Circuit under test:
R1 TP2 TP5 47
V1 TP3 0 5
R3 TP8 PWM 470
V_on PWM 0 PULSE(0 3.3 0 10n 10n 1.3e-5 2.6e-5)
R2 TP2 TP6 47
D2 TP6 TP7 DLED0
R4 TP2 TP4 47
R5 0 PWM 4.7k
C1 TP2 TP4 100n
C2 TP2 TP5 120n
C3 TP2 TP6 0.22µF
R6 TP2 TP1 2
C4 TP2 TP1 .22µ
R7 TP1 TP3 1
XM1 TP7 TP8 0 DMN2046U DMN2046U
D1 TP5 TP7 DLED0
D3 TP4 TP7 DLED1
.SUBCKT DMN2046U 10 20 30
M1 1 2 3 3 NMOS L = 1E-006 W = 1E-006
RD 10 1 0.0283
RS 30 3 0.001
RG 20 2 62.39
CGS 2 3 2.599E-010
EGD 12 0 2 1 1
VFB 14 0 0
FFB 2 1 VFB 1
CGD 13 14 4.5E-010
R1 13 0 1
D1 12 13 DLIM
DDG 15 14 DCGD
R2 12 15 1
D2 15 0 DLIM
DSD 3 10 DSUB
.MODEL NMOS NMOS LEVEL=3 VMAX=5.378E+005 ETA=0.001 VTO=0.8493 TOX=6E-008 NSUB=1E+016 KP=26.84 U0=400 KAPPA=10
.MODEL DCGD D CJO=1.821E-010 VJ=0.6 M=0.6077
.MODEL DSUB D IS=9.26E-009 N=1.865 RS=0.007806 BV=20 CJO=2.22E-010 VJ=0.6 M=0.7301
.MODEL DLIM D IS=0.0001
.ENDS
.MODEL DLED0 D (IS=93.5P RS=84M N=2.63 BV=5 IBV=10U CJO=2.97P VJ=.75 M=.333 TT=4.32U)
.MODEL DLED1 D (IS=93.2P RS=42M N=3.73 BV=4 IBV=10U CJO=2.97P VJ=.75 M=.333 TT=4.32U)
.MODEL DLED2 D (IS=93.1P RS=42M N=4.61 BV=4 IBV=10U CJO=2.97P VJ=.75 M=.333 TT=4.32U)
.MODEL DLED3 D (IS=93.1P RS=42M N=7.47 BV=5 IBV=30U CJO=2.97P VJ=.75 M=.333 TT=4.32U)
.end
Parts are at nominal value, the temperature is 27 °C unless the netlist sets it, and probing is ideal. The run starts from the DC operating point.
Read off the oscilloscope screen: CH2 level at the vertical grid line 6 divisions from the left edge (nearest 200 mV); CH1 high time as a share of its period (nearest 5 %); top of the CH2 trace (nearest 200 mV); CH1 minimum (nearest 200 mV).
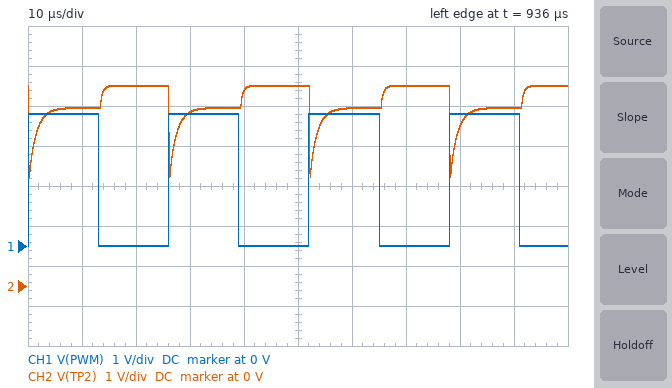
4.4 V
50 %
5.0 V
0 V
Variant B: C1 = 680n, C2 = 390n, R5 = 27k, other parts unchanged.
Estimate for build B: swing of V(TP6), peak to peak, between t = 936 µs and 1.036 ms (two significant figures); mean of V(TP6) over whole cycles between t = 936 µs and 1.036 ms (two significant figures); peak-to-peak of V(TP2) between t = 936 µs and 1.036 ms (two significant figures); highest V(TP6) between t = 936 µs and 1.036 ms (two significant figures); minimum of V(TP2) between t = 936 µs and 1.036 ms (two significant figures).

2.3 V
2.1 V
1.8 V
3.7 V
3.2 V
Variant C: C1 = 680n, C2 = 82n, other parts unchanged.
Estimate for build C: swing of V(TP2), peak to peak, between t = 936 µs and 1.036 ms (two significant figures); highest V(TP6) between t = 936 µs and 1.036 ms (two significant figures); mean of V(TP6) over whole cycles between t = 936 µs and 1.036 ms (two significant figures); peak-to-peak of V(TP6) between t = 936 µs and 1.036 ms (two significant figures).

2.1 V
4.2 V
2.3 V
2.8 V
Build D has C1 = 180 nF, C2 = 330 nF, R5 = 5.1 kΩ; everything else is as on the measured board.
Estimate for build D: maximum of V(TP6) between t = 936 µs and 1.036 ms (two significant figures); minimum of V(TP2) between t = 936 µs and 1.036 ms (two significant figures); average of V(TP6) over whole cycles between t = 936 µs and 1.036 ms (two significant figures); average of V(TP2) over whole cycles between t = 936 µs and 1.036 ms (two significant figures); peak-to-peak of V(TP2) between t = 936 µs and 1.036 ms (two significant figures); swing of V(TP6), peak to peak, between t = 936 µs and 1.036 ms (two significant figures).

4.0 V
2.9 V
2.2 V
4.6 V
2.1 V
2.6 V
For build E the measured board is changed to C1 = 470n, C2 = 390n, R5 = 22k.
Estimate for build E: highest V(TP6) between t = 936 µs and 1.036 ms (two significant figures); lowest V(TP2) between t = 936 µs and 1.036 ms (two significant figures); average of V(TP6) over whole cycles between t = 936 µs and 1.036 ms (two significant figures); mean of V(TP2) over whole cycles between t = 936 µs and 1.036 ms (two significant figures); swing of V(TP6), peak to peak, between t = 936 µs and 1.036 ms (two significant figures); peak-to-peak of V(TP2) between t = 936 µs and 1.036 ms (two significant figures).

3.8 V
3.1 V
2.1 V
4.6 V
2.4 V
1.9 V
